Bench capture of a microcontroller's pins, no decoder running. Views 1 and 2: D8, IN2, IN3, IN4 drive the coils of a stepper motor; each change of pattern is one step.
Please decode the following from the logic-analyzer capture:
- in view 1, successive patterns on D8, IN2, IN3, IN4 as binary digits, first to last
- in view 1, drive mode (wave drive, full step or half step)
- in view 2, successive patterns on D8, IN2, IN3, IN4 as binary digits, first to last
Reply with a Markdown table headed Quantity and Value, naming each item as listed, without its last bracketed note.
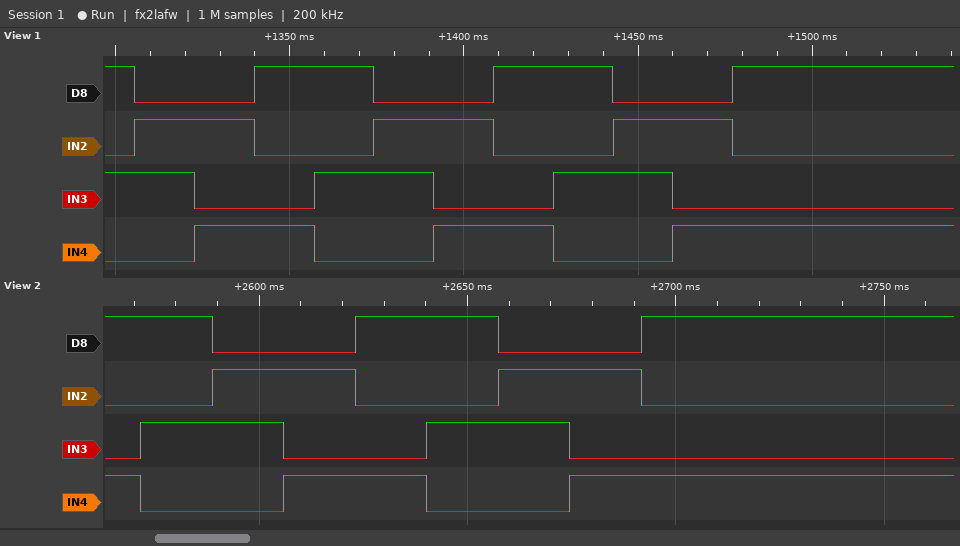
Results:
| Quantity | Value |
|---|---|
| in view 1, successive patterns on D8, IN2, IN3, IN4 as binary digits, first to last | 1010 0110 0101 1001 1010 0110 0101 1001 1010 0110 0101 1001 |
| in view 1, drive mode | full step |
| in view 2, successive patterns on D8, IN2, IN3, IN4 as binary digits, first to last | 1001 1010 0110 0101 1001 1010 0110 0101 1001 |
